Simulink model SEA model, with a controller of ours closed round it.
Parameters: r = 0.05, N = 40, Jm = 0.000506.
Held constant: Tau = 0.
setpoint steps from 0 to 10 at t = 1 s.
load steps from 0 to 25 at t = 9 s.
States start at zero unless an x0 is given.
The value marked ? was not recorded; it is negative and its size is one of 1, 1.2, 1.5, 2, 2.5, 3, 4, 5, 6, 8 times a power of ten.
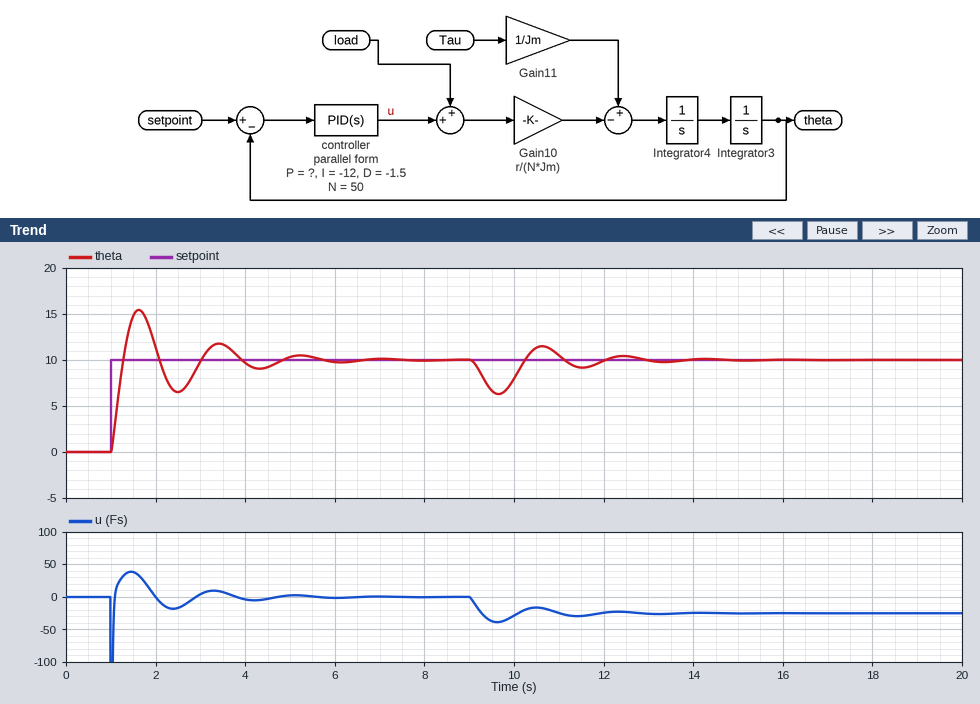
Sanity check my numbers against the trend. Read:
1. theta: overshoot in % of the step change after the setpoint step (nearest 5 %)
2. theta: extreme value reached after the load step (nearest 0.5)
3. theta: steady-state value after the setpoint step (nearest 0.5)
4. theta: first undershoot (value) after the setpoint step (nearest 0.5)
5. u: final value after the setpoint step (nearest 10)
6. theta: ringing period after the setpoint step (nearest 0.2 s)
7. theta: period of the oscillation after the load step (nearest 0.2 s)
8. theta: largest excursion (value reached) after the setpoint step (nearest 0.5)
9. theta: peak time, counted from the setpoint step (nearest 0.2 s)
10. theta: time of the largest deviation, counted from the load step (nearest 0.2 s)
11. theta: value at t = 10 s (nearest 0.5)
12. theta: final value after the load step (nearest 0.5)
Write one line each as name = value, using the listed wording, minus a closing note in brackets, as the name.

theta: overshoot in % of the step change after the setpoint step = 55 %
theta: extreme value reached after the load step = 6.5
theta: steady-state value after the setpoint step = 10.0
theta: first undershoot (value) after the setpoint step = 6.5
u: final value after the setpoint step = 0
theta: ringing period after the setpoint step = 1.8 s
theta: period of the oscillation after the load step = 1.8 s
theta: largest excursion (value reached) after the setpoint step = 15.5
theta: peak time, counted from the setpoint step = 0.6 s
theta: time of the largest deviation, counted from the load step = 0.6 s
theta: value at t = 10 s = 8.0
theta: final value after the load step = 10.0
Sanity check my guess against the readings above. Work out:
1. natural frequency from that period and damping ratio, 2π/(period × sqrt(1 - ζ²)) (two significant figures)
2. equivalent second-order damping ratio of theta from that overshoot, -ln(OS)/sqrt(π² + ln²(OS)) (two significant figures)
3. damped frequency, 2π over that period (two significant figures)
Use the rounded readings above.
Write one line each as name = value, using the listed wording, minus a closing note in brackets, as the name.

natural frequency from that period and damping ratio, 2π/(period × sqrt(1 - ζ²)) = 3.6 rad/s
equivalent second-order damping ratio of theta from that overshoot, -ln(OS)/sqrt(π² + ln²(OS)) = 0.19
damped frequency, 2π over that period = 3.5 rad/s
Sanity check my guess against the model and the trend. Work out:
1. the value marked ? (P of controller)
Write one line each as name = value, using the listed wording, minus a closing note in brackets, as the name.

the value marked ? = -6
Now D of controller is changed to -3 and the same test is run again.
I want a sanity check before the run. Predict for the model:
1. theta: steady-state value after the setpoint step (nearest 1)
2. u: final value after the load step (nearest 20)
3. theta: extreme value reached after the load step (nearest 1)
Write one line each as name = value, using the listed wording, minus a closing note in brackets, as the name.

theta: steady-state value after the setpoint step = 10
u: final value after the load step = -20
theta: extreme value reached after the load step = 7
